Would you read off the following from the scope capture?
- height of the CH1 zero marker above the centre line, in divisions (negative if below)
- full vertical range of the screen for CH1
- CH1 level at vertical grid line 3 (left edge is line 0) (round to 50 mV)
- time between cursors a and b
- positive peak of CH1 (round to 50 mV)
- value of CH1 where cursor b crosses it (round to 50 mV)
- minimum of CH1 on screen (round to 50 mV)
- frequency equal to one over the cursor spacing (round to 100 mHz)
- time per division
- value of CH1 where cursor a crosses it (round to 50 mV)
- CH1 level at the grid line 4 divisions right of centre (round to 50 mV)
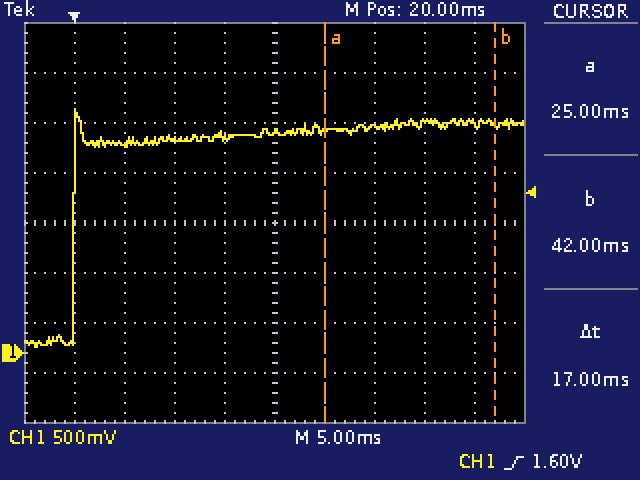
-2.6 div
4 V
2.15 V
17 ms
2.45 V
2.30 V
50 mV
58.8 Hz
5 ms
2.20 V
2.30 V
